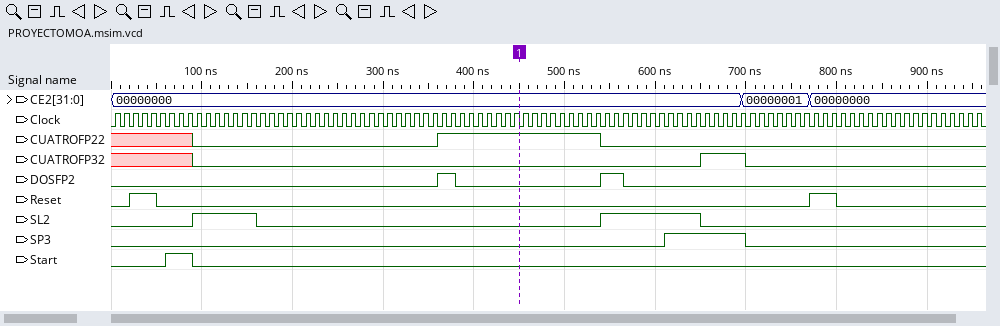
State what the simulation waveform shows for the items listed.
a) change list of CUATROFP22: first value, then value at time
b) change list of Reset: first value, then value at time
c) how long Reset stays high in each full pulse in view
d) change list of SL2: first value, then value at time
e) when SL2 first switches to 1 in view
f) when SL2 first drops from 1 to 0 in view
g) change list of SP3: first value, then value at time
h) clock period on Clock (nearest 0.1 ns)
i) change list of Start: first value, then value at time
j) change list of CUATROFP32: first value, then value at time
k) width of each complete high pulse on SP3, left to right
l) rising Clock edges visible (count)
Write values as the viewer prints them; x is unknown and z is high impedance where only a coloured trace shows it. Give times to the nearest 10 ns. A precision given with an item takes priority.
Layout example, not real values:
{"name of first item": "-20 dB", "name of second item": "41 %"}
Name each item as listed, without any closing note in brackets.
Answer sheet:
{"change list of CUATROFP22: first value, then value at time": "x, 0 at 90 ns, 1 at 360 ns, 0 at 540 ns", "change list of Reset: first value, then value at time": "0, 1 at 20 ns, 0 at 50 ns, 1 at 770 ns, 0 at 800 ns", "how long Reset stays high in each full pulse in view": "30 ns, 30 ns", "change list of SL2: first value, then value at time": "0, 1 at 90 ns, 0 at 160 ns, 1 at 540 ns, 0 at 650 ns", "when SL2 first switches to 1 in view": "90 ns", "when SL2 first drops from 1 to 0 in view": "160 ns", "change list of SP3: first value, then value at time": "0, 1 at 610 ns, 0 at 700 ns", "clock period on Clock": "10 ns", "change list of Start: first value, then value at time": "0, 1 at 60 ns, 0 at 90 ns", "change list of CUATROFP32: first value, then value at time": "x, 0 at 90 ns, 1 at 650 ns, 0 at 700 ns", "width of each complete high pulse on SP3, left to right": "90 ns", "rising Clock edges visible": "96"}
